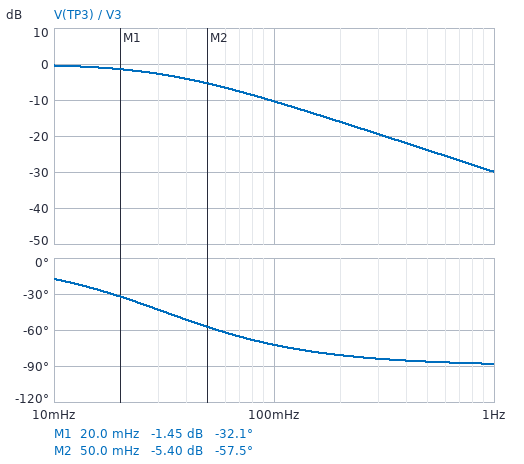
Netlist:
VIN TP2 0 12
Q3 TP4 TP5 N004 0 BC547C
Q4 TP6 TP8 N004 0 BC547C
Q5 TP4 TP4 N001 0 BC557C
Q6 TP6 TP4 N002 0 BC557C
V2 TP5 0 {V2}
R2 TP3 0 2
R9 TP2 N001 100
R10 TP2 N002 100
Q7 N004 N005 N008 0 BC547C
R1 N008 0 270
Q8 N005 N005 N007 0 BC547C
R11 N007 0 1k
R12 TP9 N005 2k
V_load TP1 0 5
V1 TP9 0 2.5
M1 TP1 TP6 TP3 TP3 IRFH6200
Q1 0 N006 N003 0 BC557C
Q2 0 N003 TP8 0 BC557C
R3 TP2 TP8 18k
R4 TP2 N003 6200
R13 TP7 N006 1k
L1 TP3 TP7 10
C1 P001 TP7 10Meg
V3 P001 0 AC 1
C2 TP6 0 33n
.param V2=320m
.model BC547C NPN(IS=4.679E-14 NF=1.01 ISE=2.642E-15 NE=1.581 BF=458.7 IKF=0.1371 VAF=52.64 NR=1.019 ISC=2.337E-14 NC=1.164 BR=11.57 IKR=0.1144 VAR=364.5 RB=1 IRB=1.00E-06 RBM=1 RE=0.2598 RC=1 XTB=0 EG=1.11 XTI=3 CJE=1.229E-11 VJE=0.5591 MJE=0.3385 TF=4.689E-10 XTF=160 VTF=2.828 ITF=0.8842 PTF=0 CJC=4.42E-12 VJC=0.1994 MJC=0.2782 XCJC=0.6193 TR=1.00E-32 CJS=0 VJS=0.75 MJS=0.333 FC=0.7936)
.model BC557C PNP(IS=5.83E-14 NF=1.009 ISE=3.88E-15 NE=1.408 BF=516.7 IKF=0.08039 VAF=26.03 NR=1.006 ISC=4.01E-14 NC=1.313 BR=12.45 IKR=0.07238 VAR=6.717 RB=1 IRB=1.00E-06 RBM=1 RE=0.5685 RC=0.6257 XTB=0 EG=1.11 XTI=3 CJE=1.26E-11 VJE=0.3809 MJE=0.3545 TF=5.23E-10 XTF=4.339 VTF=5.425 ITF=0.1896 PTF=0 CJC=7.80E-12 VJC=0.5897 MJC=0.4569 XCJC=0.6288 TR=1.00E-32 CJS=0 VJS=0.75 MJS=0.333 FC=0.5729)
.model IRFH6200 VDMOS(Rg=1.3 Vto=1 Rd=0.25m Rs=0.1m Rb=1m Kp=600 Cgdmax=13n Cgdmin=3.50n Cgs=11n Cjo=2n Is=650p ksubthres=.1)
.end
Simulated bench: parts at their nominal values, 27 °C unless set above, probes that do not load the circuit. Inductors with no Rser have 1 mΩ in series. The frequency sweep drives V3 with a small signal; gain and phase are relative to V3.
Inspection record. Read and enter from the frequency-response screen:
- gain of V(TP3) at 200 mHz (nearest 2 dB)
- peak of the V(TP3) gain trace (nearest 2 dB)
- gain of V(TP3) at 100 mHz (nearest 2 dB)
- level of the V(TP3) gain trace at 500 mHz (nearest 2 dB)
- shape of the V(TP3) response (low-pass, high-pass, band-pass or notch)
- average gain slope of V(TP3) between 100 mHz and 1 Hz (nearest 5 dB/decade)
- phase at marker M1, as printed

-16 dB
0 dB
-10 dB
-24 dB
low-pass
-20 dB/decade
-32.1 deg
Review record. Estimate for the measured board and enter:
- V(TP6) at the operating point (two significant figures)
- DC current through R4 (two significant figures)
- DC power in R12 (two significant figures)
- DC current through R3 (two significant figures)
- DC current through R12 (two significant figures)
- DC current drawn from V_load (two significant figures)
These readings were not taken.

280 mV
1.8 mA
1.2 mW
610 µA
780 µA
1.7 µA
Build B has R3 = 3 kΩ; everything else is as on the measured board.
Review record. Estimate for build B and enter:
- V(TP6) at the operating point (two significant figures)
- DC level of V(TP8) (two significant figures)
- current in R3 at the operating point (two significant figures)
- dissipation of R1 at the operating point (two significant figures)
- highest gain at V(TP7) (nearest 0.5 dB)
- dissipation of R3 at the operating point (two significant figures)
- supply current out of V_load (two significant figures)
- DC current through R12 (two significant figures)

570 mV
1.3 V
3.6 mA
1.1 mW
0 dB
38 mW
510 µA
660 µA
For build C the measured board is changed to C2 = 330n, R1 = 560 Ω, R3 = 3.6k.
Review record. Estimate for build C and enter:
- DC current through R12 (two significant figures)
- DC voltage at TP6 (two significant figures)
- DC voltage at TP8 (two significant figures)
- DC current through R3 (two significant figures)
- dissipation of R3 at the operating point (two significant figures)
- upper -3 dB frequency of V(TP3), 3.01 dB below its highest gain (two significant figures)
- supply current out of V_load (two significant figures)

650 µA
590 mV
1.3 V
3.0 mA
32 mW
31 mHz
830 µA
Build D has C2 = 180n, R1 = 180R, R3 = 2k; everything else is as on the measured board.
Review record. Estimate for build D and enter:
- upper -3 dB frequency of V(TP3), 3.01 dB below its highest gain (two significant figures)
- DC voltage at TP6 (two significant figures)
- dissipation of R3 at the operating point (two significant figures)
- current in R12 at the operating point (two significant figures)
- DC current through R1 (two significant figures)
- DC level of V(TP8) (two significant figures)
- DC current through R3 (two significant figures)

31 mHz
570 mV
57 mW
660 µA
2.9 mA
1.3 V
5.4 mA
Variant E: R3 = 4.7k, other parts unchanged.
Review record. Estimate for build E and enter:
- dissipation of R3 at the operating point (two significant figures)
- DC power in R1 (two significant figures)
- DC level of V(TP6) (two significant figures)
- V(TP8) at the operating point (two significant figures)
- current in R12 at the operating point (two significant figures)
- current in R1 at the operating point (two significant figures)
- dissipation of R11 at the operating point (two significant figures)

25 mW
970 µW
540 mV
1.2 V
670 µA
1.9 mA
310 µW
